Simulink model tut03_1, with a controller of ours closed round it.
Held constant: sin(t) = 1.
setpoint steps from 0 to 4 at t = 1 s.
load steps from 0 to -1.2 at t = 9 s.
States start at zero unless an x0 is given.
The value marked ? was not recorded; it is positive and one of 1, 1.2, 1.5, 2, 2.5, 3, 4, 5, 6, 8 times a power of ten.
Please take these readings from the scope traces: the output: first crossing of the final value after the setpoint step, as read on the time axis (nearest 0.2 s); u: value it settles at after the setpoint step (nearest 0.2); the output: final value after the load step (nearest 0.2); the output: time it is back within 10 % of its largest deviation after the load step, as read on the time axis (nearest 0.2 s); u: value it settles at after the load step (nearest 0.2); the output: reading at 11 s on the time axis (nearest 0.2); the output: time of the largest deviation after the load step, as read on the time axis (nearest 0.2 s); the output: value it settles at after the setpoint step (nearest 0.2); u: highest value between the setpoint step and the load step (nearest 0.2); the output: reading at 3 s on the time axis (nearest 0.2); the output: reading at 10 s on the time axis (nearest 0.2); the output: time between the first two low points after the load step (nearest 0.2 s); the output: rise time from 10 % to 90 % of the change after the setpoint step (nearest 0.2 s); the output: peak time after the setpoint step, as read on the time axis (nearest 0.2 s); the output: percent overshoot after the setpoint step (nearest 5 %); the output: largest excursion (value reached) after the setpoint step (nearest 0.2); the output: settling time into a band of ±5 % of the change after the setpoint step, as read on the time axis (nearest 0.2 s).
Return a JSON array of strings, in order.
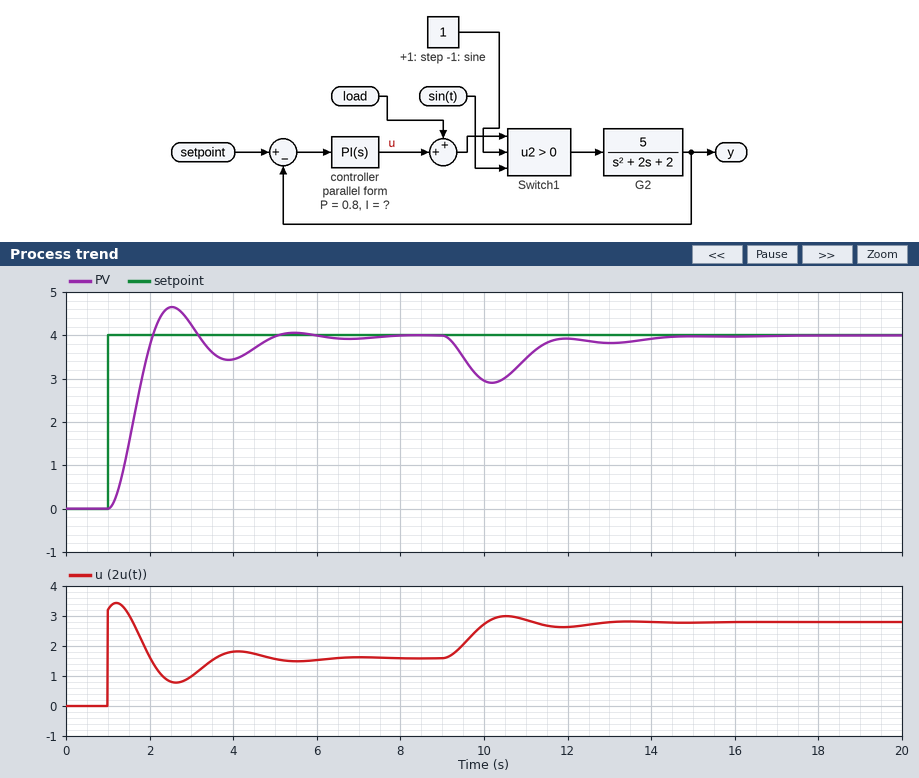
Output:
["2.0 s", "1.6", "4.0", "13.8 s", "2.8", "3.4", "10.2 s", "4.0", "3.4", "4.2", "3.0", "2.8 s", "0.8 s", "2.6 s", "15 %", "4.6", "4.6 s"]
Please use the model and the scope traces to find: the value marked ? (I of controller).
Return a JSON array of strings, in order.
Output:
["0.6"]
